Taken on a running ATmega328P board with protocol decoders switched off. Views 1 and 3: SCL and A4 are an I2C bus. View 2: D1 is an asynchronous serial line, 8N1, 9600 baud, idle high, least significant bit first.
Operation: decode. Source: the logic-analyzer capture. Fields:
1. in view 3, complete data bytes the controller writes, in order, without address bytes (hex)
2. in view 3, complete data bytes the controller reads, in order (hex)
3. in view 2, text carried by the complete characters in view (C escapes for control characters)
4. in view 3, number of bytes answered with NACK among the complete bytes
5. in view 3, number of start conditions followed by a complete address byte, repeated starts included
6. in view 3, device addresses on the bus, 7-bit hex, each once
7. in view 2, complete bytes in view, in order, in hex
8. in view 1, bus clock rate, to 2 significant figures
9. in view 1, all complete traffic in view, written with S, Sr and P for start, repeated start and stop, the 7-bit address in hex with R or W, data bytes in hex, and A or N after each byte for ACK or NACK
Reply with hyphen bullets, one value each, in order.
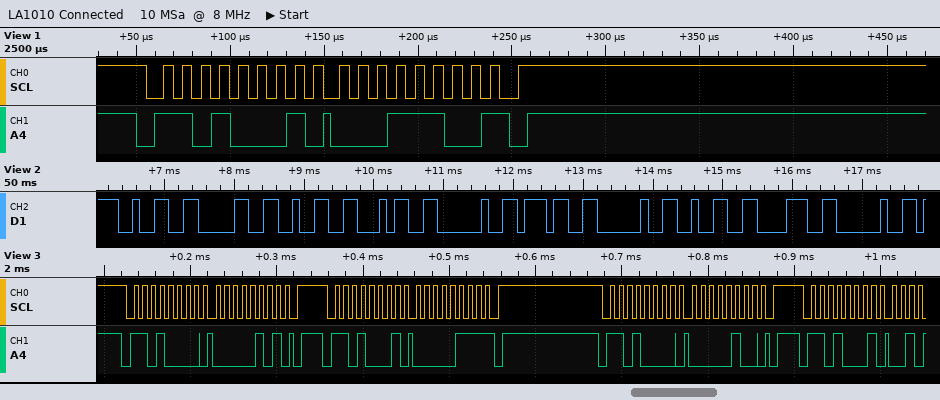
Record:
- 05 04
- 07
- "2024 7 28 "
- 1
- 4
- 0x68
- 32 30 32 34 20 37 20 32 38 20
- 100 kHz
- S 68R A 1C N P
